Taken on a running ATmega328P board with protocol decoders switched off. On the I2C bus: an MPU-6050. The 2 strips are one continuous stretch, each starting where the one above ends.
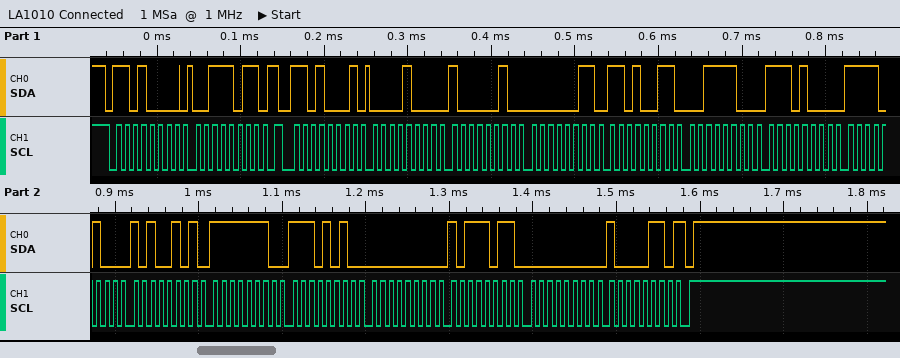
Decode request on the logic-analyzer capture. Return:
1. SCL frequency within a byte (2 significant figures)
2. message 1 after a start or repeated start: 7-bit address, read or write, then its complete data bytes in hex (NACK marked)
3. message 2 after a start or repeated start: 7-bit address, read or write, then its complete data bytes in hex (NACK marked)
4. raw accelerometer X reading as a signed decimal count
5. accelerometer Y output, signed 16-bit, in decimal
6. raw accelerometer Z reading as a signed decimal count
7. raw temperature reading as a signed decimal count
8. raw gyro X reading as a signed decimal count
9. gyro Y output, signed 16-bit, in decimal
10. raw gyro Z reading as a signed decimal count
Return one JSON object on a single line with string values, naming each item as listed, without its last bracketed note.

{"SCL frequency within a byte": "100 kHz", "message 1 after a start or repeated start: 7-bit address, read or write, then its complete data bytes in hex": "0x68 write: 3B", "message 2 after a start or repeated start: 7-bit address, read or write, then its complete data bytes in hex": "0x68 read: 08 82 03 D3 3C E8 F4 A5 FE EA 00 BB 00 86 NACK", "raw accelerometer X reading as a signed decimal count": "2178", "accelerometer Y output, signed 16-bit, in decimal": "979", "raw accelerometer Z reading as a signed decimal count": "15592", "raw temperature reading as a signed decimal count": "-2907", "raw gyro X reading as a signed decimal count": "-278", "gyro Y output, signed 16-bit, in decimal": "187", "raw gyro Z reading as a signed decimal count": "134"}
